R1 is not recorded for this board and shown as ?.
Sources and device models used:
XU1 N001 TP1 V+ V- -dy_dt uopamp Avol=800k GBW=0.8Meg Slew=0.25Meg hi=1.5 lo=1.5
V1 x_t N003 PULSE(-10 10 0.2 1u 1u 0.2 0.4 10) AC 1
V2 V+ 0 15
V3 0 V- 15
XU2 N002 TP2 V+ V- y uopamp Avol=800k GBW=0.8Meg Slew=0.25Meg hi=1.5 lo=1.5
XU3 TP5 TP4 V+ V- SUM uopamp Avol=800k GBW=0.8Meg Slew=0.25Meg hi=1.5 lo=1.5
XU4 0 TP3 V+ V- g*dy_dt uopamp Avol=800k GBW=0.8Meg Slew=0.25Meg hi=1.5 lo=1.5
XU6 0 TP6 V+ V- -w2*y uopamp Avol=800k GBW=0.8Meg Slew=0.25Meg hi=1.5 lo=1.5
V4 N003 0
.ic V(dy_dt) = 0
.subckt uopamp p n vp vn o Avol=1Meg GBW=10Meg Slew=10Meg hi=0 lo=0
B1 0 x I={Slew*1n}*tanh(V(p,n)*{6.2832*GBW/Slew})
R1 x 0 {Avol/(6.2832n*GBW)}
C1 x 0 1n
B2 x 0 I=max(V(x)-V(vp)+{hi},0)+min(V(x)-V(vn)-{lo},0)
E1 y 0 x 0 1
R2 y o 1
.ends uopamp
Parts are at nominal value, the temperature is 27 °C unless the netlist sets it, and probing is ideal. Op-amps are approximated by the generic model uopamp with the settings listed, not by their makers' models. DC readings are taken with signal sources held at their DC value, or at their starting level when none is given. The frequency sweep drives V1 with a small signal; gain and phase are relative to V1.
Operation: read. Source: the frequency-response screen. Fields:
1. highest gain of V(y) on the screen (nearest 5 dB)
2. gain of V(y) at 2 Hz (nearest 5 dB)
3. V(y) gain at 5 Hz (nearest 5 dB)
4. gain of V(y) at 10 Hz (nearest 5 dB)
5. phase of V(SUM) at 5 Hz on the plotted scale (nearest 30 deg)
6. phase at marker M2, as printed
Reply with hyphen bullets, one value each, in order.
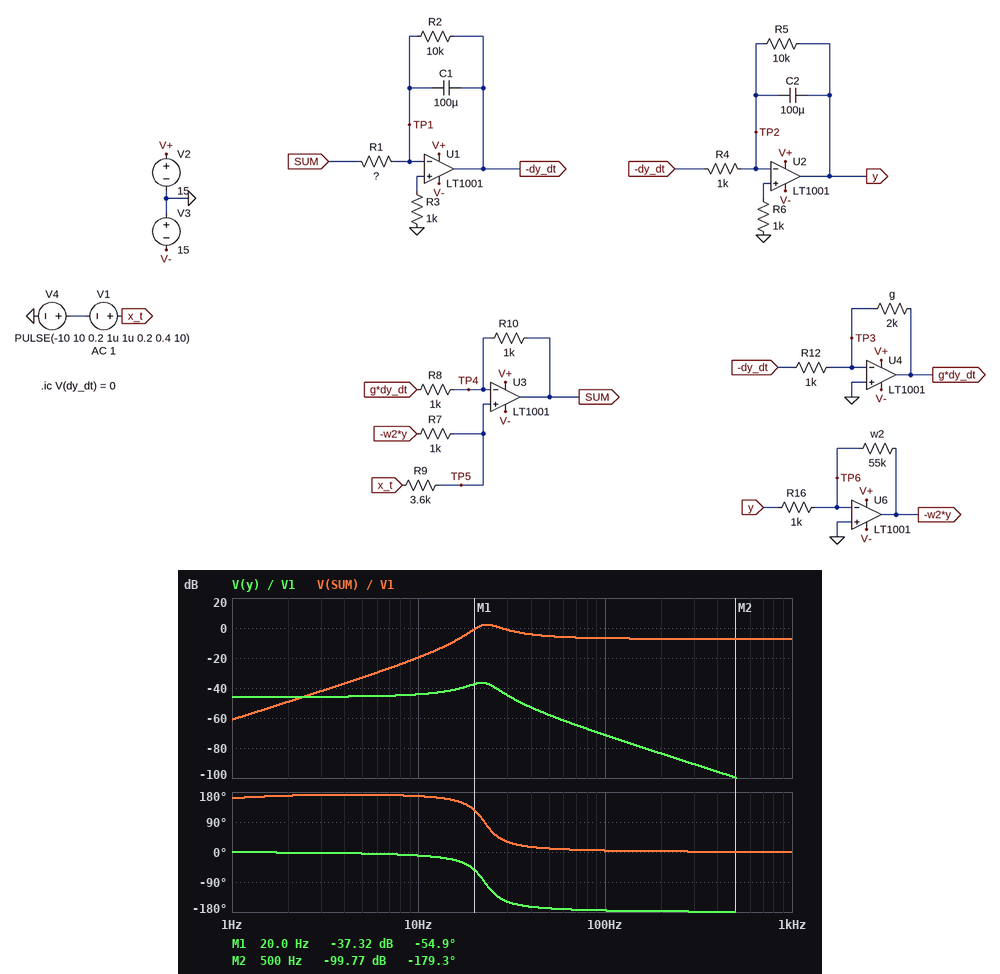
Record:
- -35 dB
- -45 dB
- -45 dB
- -45 dB
- 180 deg
- -179.3 deg
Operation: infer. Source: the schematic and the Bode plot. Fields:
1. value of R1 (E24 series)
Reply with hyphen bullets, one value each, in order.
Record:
- 430 Ω
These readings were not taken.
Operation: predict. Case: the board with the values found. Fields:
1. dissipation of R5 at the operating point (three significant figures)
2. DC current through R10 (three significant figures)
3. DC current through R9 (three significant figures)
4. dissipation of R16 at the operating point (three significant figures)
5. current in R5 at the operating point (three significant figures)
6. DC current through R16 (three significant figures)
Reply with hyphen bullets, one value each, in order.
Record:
- 254 nW
- 4.93 µA
- 2.78 mA
- 2.54 µW
- 5.04 µA
- 50.4 µA
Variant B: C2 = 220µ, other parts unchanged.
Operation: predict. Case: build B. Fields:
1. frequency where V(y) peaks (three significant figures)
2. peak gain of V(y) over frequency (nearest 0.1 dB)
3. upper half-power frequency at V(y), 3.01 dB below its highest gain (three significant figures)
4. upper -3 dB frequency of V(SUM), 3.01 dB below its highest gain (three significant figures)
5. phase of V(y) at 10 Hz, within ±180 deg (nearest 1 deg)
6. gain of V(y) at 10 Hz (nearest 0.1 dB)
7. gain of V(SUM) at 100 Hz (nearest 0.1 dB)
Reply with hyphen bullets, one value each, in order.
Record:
- 14.2 Hz
- -39.7 dB
- 17.7 Hz
- 24.4 Hz
- -30 deg
- -42.3 dB
- -7.1 dB
